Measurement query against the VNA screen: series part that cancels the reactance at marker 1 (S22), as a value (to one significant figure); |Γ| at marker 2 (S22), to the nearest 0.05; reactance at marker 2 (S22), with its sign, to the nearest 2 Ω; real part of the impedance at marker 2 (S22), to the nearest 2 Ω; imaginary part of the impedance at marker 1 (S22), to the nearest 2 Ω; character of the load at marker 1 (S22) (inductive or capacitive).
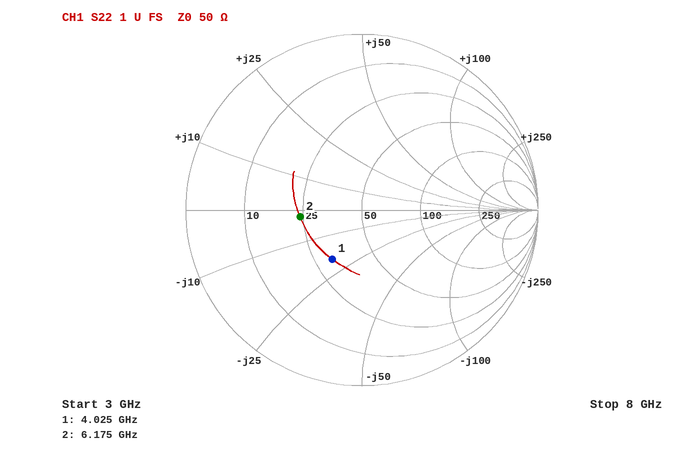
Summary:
800 pH
0.35
-2 Ω
24 Ω
-20 Ω
capacitive
